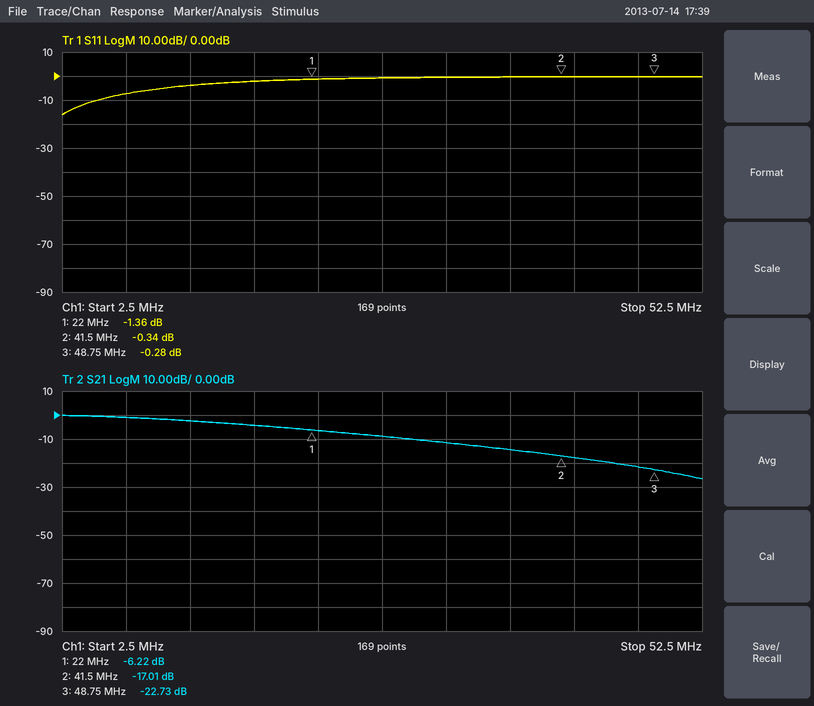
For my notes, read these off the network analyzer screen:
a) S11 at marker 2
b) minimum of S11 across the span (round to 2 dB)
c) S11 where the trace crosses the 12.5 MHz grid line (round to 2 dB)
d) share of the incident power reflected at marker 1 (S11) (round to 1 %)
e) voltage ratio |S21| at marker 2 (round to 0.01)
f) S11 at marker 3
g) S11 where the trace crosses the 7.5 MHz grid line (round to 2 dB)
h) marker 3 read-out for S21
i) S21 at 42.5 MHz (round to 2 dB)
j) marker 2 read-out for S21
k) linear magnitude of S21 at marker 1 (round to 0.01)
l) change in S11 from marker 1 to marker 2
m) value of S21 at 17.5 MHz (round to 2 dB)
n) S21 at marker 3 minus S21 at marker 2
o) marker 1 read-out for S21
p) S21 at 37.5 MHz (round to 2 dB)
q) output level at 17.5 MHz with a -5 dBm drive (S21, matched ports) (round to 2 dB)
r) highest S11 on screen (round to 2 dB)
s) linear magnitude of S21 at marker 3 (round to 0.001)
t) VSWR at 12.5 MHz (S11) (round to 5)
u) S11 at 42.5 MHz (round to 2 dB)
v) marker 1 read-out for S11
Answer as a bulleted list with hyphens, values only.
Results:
- -0.34 dB
- -16 dB
- -4 dB
- 73 %
- 0.14
- -0.28 dB
- -8 dB
- -22.73 dB
- -18 dB
- -17.01 dB
- 0.49
- 1.02 dB
- -4 dB
- -5.72 dB
- -6.22 dB
- -14 dB
- -10 dBm
- 0 dB
- 0.073
- 5
- 0 dB
- -1.36 dB
